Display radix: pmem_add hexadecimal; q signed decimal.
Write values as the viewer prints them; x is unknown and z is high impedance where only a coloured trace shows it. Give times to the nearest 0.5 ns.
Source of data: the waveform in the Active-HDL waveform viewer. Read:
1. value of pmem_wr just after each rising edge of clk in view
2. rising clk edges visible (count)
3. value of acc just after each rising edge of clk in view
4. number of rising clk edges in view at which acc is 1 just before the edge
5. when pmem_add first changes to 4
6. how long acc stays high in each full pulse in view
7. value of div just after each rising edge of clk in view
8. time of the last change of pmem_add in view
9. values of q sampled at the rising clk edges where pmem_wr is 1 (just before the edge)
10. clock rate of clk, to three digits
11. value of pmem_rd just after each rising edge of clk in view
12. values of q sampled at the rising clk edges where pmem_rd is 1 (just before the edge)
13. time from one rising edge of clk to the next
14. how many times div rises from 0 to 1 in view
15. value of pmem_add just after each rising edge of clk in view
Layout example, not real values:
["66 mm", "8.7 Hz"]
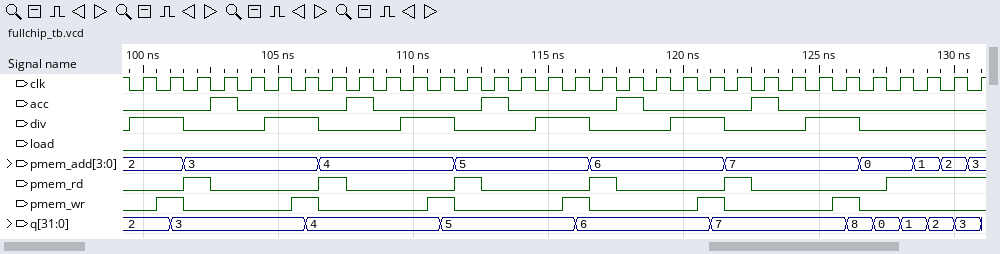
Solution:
["0 1 0 0 0 0 1 0 0 0 0 1 0 0 0 0 1 0 0 0 0 1 0 0 0 0 1 0 0 0 0 0", "32", "0 0 0 1 0 0 0 0 1 0 0 0 0 1 0 0 0 0 1 0 0 0 0 1 0 0 0 0 0 0 0 0", "5", "106.5 ns", "1 ns, 1 ns, 1 ns, 1 ns, 1 ns", "1 1 0 0 0 1 1 0 0 0 1 1 0 0 0 1 1 0 0 0 1 1 0 0 0 1 1 0 0 0 0 0", "130.5 ns", "2, 3, 4, 5, 6, 7", "1.00 GHz", "0 0 1 0 0 0 0 1 0 0 0 0 1 0 0 0 0 1 0 0 0 0 1 0 0 0 0 0 1 1 1 1", "3, 4, 5, 6, 7, 0, 1, 2, 3", "1 ns", "6", "2, 2, 3, 3, 3, 3, 3, 4, 4, 4, 4, 4, 5, 5, 5, 5, 5, 6, 6, 6, 6, 6, 7, 7, 7, 7, 7, 0, 0, 1, 2, 3"]
